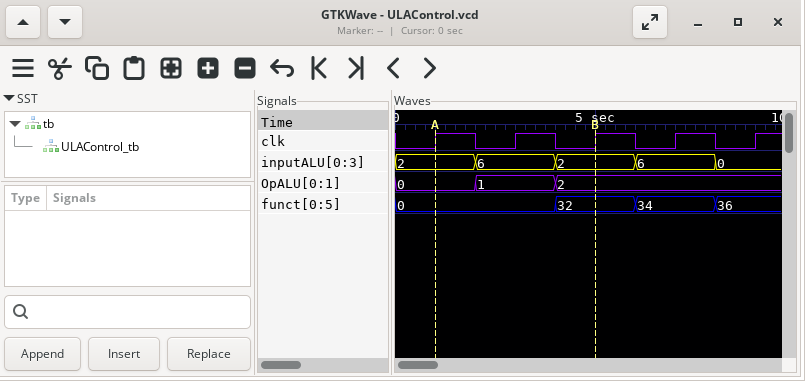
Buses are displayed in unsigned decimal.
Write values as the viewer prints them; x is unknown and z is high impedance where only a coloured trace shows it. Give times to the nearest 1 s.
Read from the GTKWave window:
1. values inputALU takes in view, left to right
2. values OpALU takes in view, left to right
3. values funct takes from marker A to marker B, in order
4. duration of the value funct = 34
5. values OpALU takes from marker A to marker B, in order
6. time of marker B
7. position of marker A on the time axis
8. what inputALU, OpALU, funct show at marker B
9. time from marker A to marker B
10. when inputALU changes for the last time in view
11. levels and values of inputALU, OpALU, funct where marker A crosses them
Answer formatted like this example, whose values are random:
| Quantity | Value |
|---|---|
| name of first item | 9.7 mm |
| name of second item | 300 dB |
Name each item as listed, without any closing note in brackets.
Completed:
| Quantity | Value |
|---|---|
| values inputALU takes in view, left to right | 2, 6, 2, 6, 0 |
| values OpALU takes in view, left to right | 0, 1, 2 |
| values funct takes from marker A to marker B, in order | 0, 32 |
| duration of the value funct = 34 | 2 s |
| values OpALU takes from marker A to marker B, in order | 0, 1, 2 |
| time of marker B | 5 s |
| position of marker A on the time axis | 1 s |
| what inputALU, OpALU, funct show at marker B | inputALU=2, OpALU=2, funct=32 |
| time from marker A to marker B | 4 s |
| when inputALU changes for the last time in view | 8 s |
| levels and values of inputALU, OpALU, funct where marker A crosses them | inputALU=2, OpALU=0, funct=0 |
